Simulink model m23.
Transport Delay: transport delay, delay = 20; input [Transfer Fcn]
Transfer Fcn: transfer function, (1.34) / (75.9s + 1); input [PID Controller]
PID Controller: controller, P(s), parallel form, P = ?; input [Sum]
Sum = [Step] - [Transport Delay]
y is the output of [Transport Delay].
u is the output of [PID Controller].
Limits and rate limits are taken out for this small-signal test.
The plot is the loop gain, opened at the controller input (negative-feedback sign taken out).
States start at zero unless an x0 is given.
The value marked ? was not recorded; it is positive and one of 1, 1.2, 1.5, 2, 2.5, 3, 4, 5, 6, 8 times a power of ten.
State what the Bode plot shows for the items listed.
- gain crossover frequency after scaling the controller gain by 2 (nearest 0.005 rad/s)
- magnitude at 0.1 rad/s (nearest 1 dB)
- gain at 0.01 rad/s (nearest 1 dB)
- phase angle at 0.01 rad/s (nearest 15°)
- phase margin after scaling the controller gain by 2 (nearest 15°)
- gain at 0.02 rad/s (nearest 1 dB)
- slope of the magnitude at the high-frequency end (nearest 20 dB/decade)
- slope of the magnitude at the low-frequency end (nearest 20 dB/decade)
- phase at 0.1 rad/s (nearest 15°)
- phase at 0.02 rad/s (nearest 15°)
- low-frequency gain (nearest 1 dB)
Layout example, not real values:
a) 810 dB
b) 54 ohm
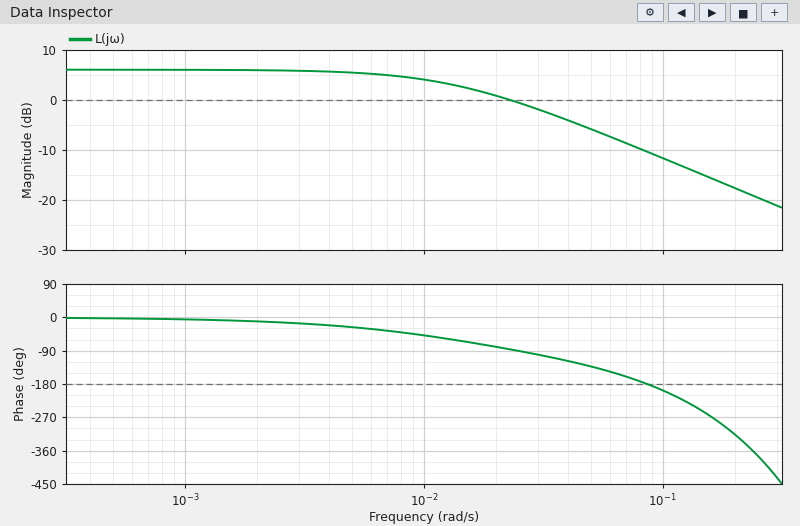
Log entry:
a) 0.050 rad/s
b) -12 dB
c) 4 dB
d) -45°
e) 45°
f) 1 dB
g) -20 dB/decade
h) 0 dB/decade
i) -195°
j) -75°
k) 6 dB
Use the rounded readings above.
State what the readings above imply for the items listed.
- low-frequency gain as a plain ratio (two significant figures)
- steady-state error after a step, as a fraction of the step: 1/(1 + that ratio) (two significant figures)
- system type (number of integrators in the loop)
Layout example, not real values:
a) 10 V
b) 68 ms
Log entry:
a) 2.0
b) 0.33
c) 0
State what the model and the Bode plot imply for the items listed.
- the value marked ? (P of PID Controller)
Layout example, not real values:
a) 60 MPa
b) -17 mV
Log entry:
a) 1.5
